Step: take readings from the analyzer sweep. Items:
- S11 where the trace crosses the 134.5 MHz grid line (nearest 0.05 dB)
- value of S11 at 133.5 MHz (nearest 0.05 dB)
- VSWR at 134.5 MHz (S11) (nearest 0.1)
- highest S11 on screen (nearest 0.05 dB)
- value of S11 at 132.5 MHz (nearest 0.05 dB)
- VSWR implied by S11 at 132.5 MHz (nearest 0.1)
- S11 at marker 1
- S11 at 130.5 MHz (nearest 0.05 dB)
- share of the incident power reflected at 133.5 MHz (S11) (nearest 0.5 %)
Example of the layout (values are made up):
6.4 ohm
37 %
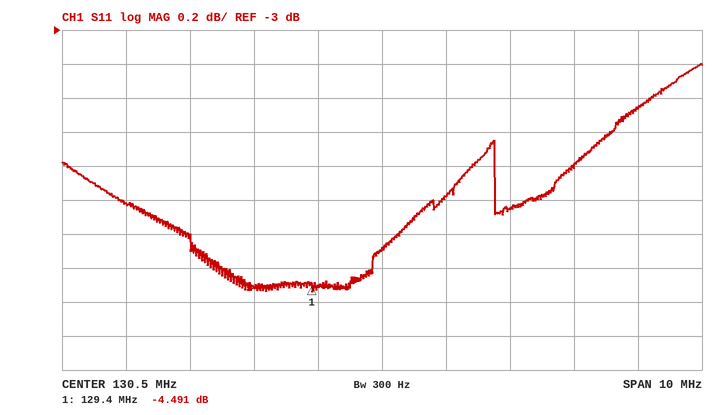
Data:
-3.45 dB
-3.80 dB
5.1
-3.20 dB
-4.05 dB
4.4
-4.491 dB
-4.30 dB
41.5 %
